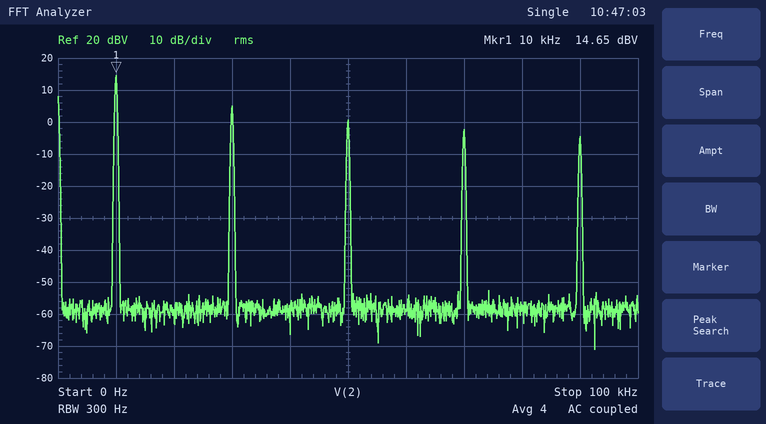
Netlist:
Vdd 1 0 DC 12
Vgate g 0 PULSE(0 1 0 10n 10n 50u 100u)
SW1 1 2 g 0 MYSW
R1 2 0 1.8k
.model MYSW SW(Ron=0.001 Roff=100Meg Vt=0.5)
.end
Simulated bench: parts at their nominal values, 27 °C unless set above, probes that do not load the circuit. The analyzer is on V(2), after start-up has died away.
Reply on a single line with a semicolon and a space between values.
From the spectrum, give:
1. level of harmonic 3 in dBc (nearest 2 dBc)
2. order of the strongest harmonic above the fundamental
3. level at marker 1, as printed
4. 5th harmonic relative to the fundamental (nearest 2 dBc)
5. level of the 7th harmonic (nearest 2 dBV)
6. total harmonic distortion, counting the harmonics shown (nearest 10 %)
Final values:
-10 dBc; 3; 14.65 dBV; -14 dBc; -2 dBV; 40 %
